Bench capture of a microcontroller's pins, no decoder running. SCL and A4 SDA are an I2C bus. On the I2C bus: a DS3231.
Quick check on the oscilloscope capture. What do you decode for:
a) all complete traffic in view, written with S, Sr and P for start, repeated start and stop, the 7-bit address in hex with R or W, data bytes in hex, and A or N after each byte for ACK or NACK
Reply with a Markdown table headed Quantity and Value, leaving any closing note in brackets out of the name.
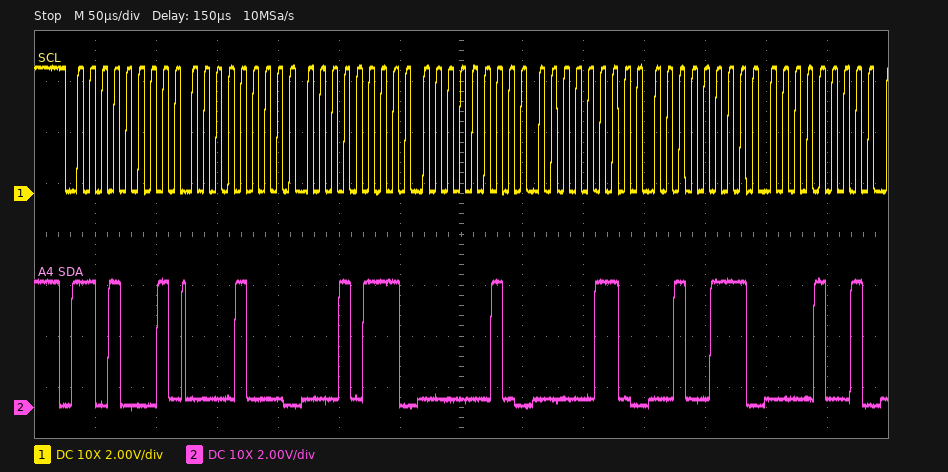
| Quantity | Value |
|---|---|
| all complete traffic in view, written with S, Sr and P for start, repeated start and stop, the 7-bit address in hex with R or W, data bytes in hex, and A or N after each byte for ACK or NACK | S 68R A 08 A 17 A 02 A 06 A 27 A 09 A |
